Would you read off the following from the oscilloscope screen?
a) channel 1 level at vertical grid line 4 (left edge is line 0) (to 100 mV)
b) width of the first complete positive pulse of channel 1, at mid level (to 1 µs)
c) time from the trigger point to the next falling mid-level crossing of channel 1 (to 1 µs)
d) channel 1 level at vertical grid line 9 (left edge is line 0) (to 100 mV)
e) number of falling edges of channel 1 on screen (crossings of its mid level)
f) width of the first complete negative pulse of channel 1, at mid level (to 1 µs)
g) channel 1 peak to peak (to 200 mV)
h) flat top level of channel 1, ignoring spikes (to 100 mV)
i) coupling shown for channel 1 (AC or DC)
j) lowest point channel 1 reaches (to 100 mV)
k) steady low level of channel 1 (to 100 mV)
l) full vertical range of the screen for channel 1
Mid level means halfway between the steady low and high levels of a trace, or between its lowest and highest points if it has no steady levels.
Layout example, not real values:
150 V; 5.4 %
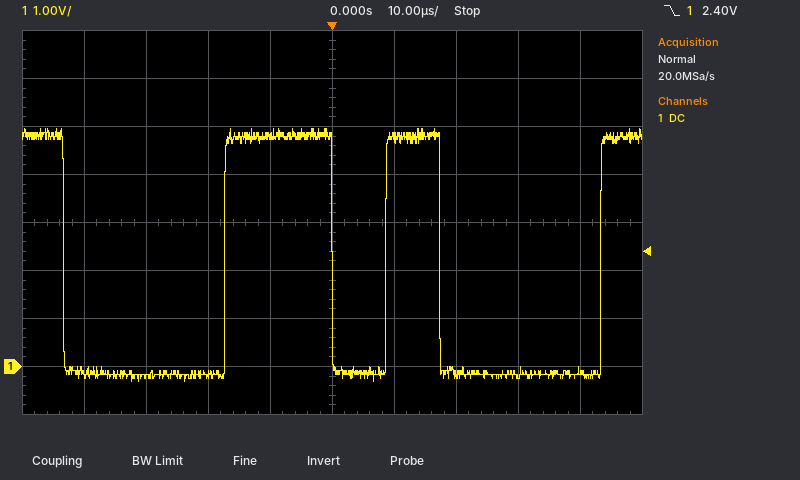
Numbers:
4.8 V; 17 µs; 17 µs; -100 mV; 3; 26 µs; 5.2 V; 4.8 V; DC; -300 mV; -200 mV; 8 V
